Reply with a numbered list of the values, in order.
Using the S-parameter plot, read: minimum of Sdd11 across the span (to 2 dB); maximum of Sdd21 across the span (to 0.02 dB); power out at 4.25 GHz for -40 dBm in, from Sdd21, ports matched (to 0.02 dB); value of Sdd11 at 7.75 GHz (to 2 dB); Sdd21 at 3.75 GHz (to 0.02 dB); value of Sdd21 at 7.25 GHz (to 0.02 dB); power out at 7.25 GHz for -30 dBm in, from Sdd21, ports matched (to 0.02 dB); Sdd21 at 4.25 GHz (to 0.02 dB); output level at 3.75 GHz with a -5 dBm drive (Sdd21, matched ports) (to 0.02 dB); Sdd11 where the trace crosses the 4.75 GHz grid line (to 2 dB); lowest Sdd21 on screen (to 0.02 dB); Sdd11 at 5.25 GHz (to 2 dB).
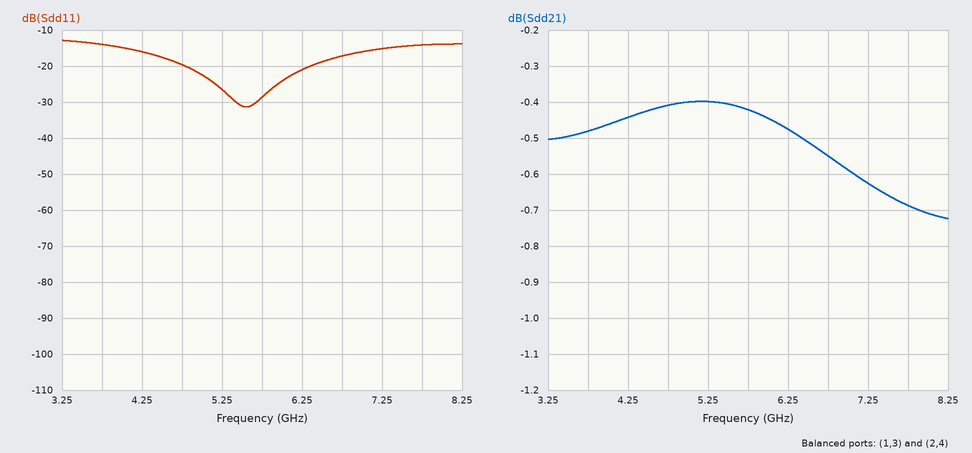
1. -32 dB
2. -0.40 dB
3. -40.44 dBm
4. -14 dB
5. -0.48 dB
6. -0.62 dB
7. -30.62 dBm
8. -0.44 dB
9. -5.48 dBm
10. -20 dB
11. -0.72 dB
12. -26 dB
